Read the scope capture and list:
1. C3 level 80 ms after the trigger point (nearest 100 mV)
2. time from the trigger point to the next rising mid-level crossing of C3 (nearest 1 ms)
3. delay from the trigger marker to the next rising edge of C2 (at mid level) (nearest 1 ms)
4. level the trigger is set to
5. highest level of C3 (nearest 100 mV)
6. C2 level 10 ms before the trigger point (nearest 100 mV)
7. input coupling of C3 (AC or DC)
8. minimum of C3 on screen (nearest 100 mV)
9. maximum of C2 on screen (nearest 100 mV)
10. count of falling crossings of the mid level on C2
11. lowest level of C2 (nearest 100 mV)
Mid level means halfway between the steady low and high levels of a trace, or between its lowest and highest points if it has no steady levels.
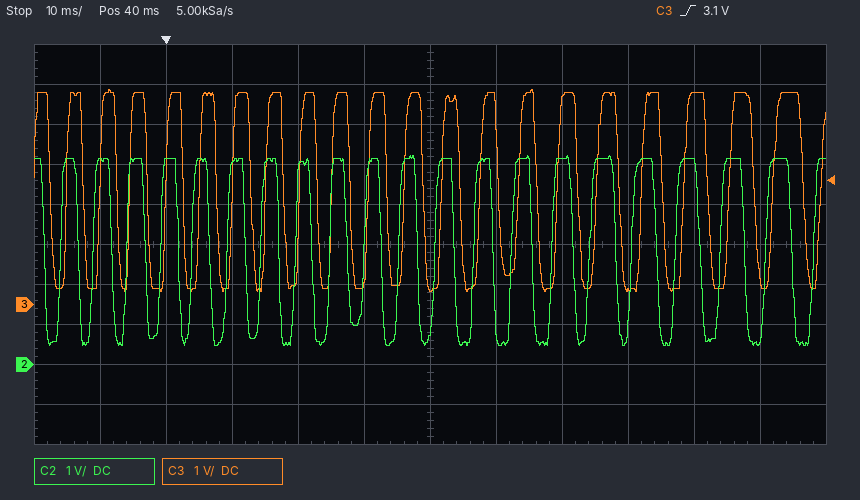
5.3 V
5 ms
4 ms
3.1 V
5.4 V
5.1 V
DC
300 mV
5.2 V
21
500 mV
